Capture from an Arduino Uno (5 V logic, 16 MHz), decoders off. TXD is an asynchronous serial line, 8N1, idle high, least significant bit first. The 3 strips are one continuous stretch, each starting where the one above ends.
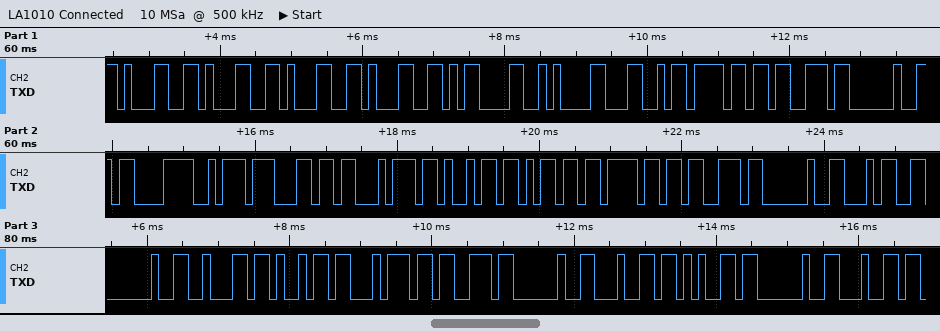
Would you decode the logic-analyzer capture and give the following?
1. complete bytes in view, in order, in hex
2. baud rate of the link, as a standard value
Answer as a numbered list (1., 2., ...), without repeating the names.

1. 31 31 31 31 0D 0A 4C 6F 73 20 C3 BA 6C 74 69 6D 6F 73 20 34 20 62 69 74 73 20 64 65 20 64
2. 9600 baud
